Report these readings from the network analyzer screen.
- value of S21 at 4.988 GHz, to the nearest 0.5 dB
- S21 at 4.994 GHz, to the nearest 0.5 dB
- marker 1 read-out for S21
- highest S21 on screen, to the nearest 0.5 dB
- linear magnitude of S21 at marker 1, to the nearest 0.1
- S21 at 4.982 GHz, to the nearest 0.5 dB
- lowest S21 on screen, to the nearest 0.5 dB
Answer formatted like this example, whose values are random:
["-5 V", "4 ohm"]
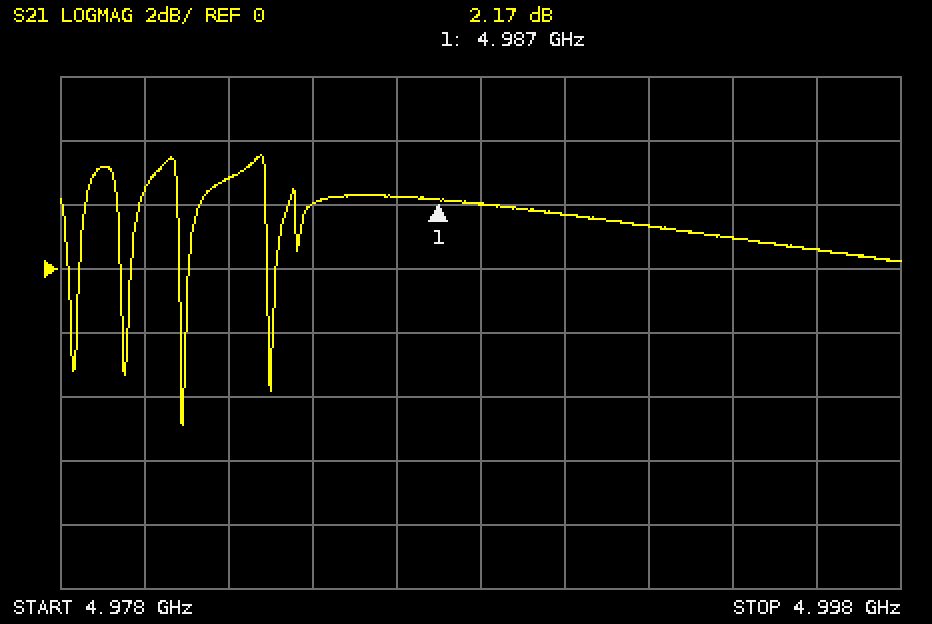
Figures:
["2.0 dB", "1.0 dB", "2.17 dB", "3.5 dB", "1.3", "3.0 dB", "-5.0 dB"]
